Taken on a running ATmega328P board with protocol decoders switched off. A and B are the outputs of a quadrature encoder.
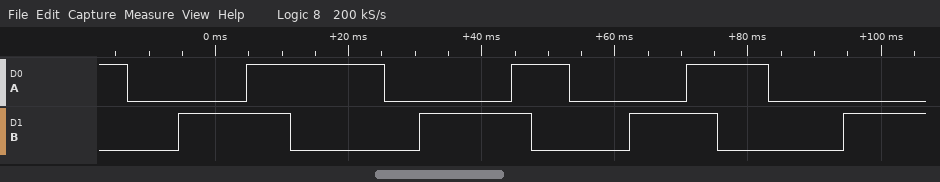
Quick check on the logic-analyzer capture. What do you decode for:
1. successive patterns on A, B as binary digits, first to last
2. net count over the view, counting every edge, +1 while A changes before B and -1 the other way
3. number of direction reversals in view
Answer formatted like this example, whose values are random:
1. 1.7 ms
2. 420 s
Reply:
1. 10 00 01 11 10 00 01 11 10 00 01 11 10 00 01
2. -14
3. 0
